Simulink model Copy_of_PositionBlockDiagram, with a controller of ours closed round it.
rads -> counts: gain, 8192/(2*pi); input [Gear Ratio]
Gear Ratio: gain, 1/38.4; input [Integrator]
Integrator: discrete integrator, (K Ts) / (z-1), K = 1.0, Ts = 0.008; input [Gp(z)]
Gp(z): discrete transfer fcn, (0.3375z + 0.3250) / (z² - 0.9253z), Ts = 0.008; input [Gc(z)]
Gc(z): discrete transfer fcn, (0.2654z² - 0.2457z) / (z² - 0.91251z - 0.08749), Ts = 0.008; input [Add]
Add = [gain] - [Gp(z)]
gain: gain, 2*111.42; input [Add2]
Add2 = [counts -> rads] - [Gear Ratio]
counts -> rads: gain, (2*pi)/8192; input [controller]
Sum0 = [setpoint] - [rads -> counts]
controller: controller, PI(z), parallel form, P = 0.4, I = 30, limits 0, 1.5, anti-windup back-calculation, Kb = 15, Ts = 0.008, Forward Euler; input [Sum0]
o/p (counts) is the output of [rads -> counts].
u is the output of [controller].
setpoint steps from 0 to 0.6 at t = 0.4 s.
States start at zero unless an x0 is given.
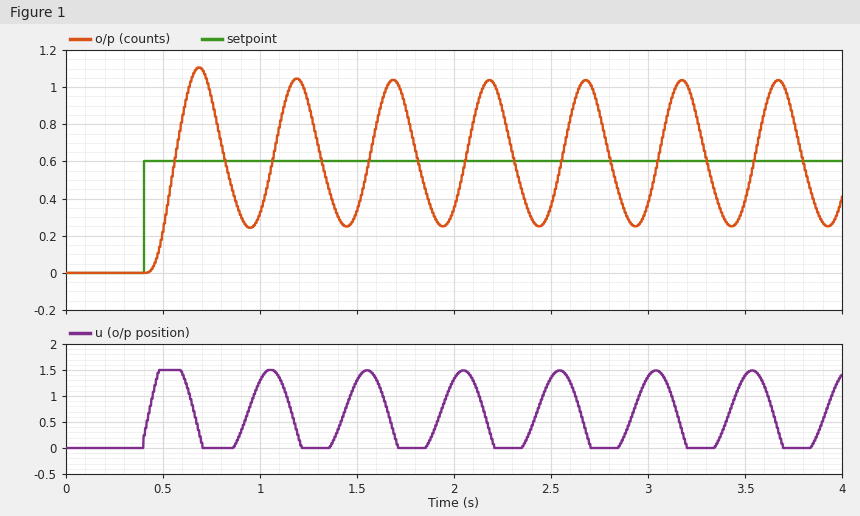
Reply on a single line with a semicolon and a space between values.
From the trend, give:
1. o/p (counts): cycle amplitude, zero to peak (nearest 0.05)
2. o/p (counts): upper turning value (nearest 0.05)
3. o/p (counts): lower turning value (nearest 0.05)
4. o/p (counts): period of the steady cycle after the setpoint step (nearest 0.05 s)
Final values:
0.40; 1.05; 0.25; 0.50 s
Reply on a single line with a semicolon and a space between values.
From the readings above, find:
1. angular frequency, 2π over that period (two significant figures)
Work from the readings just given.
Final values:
13 rad/s
